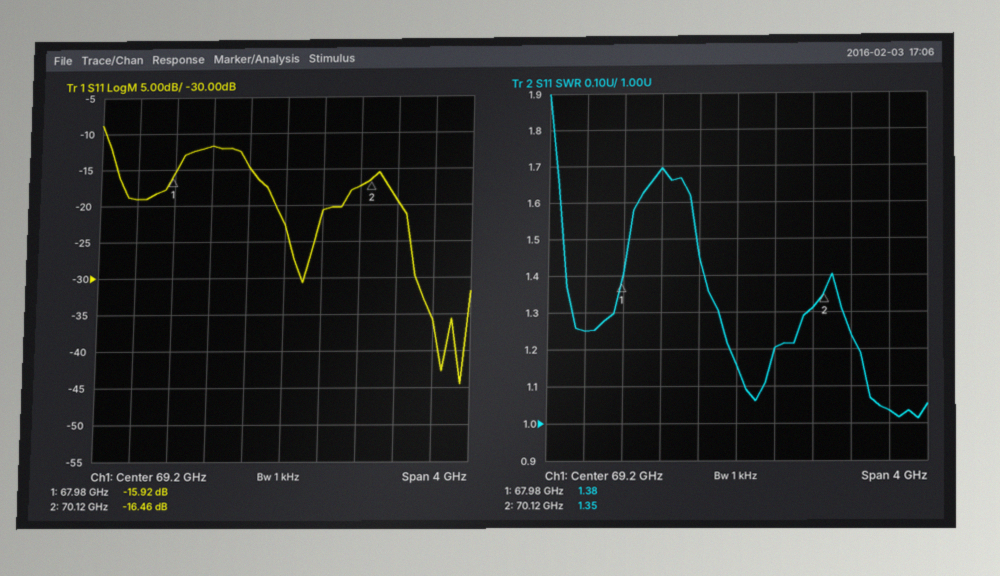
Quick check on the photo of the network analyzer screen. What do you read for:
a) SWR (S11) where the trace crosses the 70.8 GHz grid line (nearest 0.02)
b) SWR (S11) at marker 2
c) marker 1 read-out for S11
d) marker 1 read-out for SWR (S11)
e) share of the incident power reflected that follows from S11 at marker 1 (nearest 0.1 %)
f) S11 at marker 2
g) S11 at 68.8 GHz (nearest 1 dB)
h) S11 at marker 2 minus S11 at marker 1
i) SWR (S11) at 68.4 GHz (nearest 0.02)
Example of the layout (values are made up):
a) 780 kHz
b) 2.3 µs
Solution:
a) 1.04
b) 1.35
c) -15.92 dB
d) 1.38
e) 2.6 %
f) -16.46 dB
g) -15 dB
h) -0.54 dB
i) 1.70
